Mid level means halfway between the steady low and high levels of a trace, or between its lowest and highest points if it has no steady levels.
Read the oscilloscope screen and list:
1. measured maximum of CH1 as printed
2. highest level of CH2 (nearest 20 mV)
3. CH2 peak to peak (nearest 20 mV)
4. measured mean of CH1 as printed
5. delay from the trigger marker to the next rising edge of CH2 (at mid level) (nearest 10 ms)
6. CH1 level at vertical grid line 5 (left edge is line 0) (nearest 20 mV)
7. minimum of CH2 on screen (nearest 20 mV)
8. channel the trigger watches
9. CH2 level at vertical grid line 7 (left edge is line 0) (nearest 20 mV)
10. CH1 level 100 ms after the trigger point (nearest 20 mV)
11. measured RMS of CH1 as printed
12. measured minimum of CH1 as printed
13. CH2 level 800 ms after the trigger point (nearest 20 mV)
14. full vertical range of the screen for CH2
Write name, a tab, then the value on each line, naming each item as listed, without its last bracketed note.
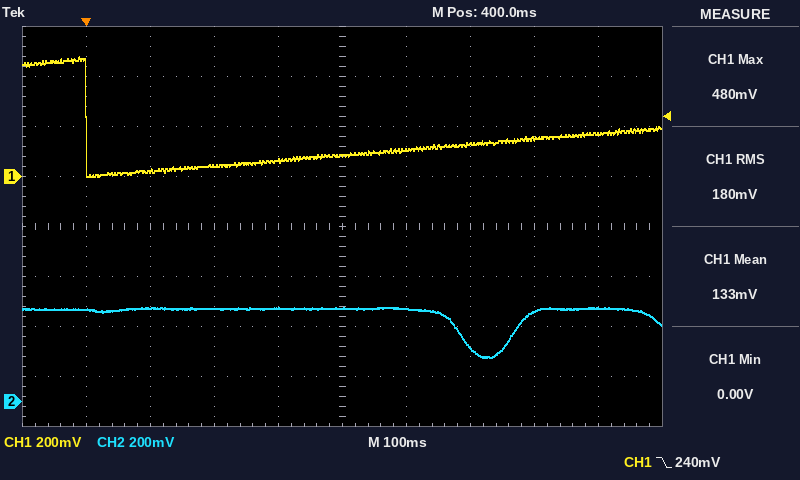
measured maximum of CH1 as printed	480 mV
highest level of CH2	380 mV
CH2 peak to peak	200 mV
measured mean of CH1 as printed	133 mV
delay from the trigger marker to the next rising edge of CH2 (at mid level)	670 ms
CH1 level at vertical grid line 5 (left edge is line 0)	80 mV
minimum of CH2 on screen	180 mV
channel the trigger watches	CH1
CH2 level at vertical grid line 7 (left edge is line 0)	220 mV
CH1 level 100 ms after the trigger point	20 mV
measured RMS of CH1 as printed	180 mV
measured minimum of CH1 as printed	0.00 V
CH2 level 800 ms after the trigger point	380 mV
full vertical range of the screen for CH2	1.6 V
